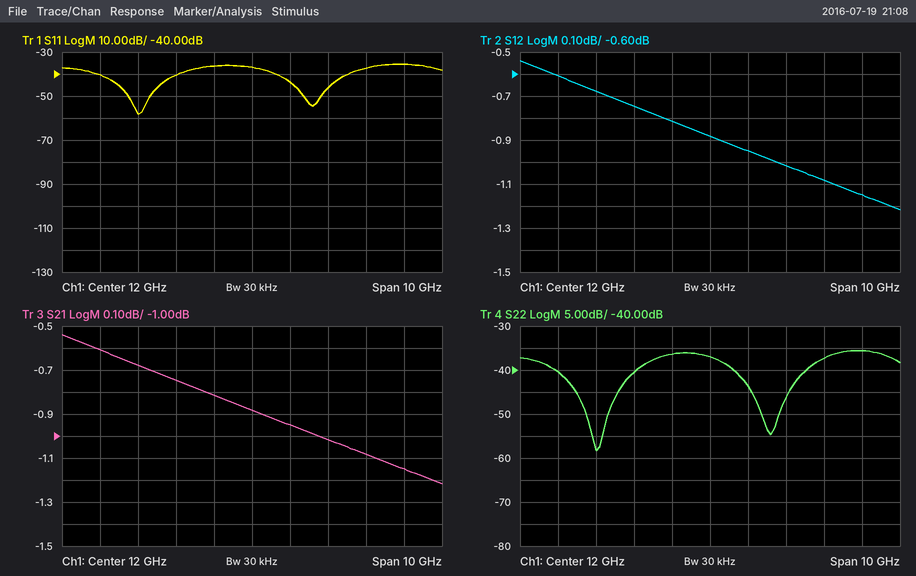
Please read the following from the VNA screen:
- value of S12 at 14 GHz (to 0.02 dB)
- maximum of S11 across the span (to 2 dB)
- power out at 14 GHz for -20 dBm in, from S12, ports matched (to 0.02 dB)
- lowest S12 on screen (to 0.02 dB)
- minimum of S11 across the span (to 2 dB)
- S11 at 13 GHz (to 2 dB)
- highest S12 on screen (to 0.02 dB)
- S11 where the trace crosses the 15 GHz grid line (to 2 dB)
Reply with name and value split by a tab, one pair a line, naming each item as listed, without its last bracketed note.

value of S12 at 14 GHz	-1.02 dB
maximum of S11 across the span	-36 dB
power out at 14 GHz for -20 dBm in, from S12, ports matched	-21.02 dBm
lowest S12 on screen	-1.22 dB
minimum of S11 across the span	-58 dB
S11 at 13 GHz	-44 dB
highest S12 on screen	-0.54 dB
S11 where the trace crosses the 15 GHz grid line	-38 dB
